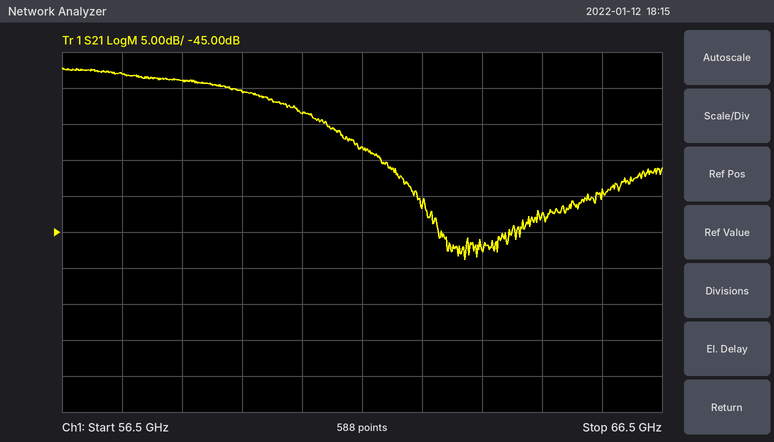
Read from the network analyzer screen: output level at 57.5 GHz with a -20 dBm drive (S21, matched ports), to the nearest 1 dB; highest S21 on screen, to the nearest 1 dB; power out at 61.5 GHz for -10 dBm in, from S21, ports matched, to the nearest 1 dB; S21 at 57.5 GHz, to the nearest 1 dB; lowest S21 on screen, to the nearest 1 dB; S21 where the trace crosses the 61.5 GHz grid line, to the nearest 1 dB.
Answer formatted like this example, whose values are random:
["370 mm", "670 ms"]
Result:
["-43 dBm", "-22 dB", "-43 dBm", "-23 dB", "-49 dB", "-33 dB"]
